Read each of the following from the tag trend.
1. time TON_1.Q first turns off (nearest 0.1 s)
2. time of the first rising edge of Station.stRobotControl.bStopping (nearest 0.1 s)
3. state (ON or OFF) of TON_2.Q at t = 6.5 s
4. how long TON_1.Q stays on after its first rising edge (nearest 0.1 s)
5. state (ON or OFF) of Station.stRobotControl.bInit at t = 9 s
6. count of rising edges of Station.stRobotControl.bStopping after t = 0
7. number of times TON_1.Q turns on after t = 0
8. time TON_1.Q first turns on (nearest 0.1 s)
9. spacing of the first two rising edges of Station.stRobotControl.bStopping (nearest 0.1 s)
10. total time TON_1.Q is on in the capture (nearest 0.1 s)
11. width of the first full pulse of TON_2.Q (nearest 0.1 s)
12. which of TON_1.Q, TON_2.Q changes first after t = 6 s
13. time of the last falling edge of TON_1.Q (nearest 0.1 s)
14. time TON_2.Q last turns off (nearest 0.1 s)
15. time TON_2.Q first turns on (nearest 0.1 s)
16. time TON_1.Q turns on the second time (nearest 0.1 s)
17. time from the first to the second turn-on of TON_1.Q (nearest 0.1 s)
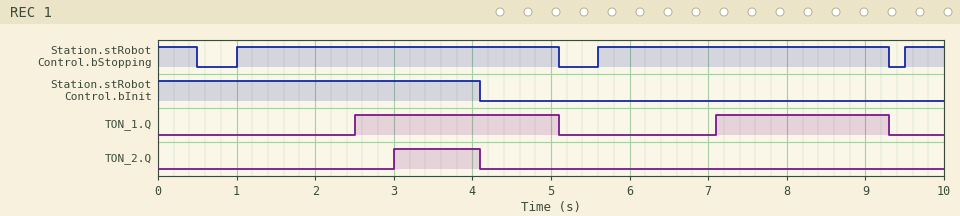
5.1 s
1.0 s
OFF
2.6 s
OFF
3
2
2.5 s
4.6 s
4.8 s
1.1 s
TON_1.Q
9.3 s
4.1 s
3.0 s
7.1 s
4.6 s
